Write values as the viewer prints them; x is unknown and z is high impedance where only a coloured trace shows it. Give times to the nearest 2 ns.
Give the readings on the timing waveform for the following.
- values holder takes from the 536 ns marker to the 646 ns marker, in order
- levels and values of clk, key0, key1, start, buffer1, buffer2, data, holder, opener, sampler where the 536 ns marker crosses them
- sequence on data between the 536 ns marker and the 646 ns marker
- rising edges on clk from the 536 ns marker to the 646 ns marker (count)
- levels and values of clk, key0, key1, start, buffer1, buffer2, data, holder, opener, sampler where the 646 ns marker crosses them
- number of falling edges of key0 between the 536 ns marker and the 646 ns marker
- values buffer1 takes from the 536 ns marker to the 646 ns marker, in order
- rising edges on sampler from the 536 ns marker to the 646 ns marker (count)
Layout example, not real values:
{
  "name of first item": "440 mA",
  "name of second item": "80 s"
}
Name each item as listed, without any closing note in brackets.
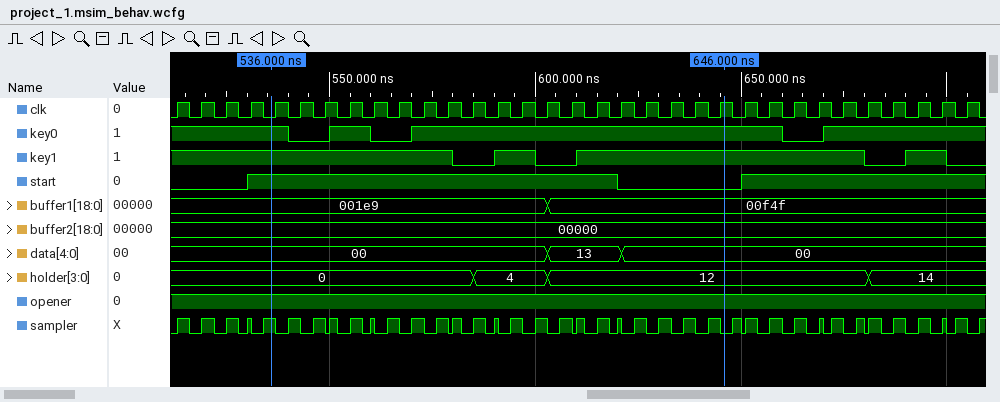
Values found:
{
  "values holder takes from the 536 ns marker to the 646 ns marker, in order": "0, 4, 12",
  "levels and values of clk, key0, key1, start, buffer1, buffer2, data, holder, opener, sampler where the 536 ns marker crosses them": "clk=0, key0=1, key1=1, start=1, buffer1=001e9, buffer2=00000, data=00, holder=0, opener=1, sampler=1",
  "sequence on data between the 536 ns marker and the 646 ns marker": "00, 13, 00",
  "rising edges on clk from the 536 ns marker to the 646 ns marker": "19",
  "levels and values of clk, key0, key1, start, buffer1, buffer2, data, holder, opener, sampler where the 646 ns marker crosses them": "clk=1, key0=1, key1=1, start=0, buffer1=00f4f, buffer2=00000, data=00, holder=12, opener=1, sampler=0",
  "number of falling edges of key0 between the 536 ns marker and the 646 ns marker": "2",
  "values buffer1 takes from the 536 ns marker to the 646 ns marker, in order": "001e9, 00f4f",
  "rising edges on sampler from the 536 ns marker to the 646 ns marker": "21"
}
